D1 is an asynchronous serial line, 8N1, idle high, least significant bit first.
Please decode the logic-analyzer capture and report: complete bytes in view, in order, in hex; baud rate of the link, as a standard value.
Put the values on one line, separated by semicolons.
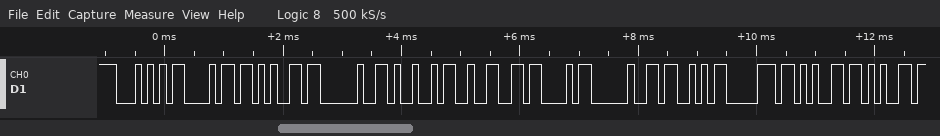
0x54 0x68 0x65 0x20 0x49 0x32 0x43 0x20 0x53 0x70 0x65 0x65; 9600 baud
